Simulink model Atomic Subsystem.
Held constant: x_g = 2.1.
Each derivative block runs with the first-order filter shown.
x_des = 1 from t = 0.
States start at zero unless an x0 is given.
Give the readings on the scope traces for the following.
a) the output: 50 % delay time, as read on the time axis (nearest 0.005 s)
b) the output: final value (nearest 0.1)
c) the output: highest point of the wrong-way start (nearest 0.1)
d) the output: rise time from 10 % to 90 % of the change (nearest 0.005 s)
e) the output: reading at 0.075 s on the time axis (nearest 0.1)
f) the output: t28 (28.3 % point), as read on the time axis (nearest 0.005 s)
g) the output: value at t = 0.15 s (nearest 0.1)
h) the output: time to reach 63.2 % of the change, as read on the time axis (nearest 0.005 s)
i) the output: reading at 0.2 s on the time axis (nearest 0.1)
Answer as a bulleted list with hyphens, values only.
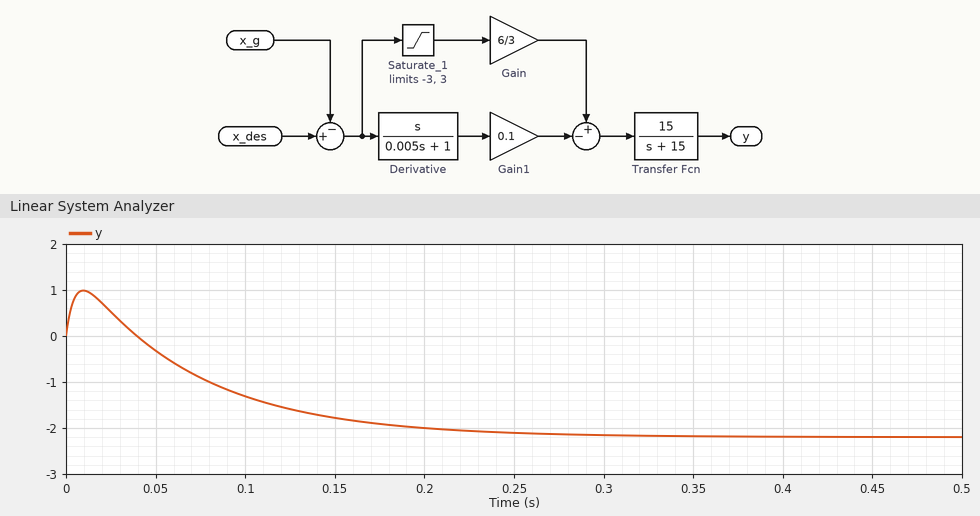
- 0.085 s
- -2.2
- 1.0
- 0.145 s
- -0.9
- 0.060 s
- -1.8
- 0.105 s
- -2.0
